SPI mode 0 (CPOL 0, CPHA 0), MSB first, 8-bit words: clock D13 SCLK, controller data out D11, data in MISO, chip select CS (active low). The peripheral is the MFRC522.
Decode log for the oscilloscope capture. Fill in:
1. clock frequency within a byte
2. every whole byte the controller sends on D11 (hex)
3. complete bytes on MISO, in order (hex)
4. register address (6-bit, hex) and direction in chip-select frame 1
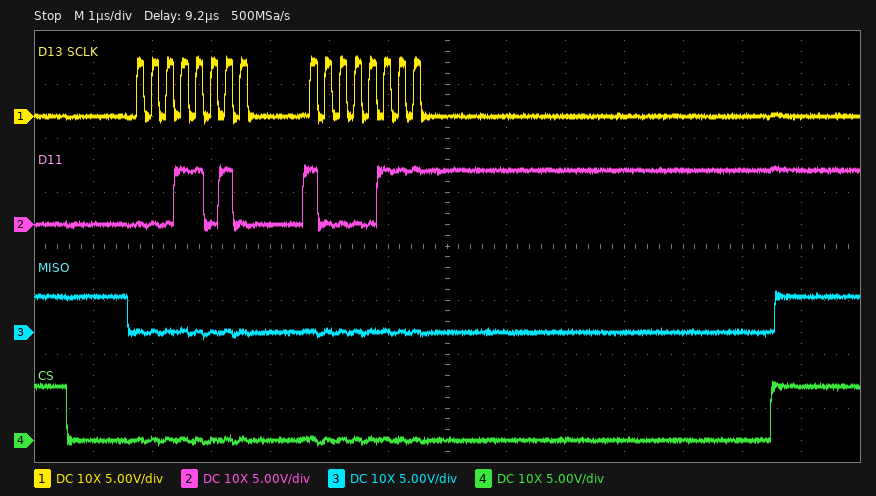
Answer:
4 MHz
0x1A 0x87
0x00 0x00
0x0D write
